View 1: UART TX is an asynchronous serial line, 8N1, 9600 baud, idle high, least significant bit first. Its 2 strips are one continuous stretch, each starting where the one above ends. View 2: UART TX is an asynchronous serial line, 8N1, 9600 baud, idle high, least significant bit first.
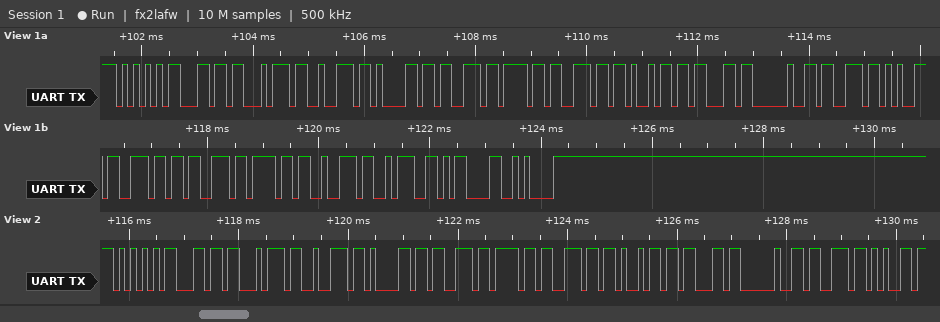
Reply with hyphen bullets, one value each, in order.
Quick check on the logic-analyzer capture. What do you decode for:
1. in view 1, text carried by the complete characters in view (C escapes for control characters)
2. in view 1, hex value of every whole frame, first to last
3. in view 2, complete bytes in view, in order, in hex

- "Ultrasonic sensor:\r\n"
- 55 6C 74 72 61 73 6F 6E 69 63 20 73 65 6E 73 6F 72 3A 0D 0A
- 0x55 0x6C 0x74 0x72 0x61 0x73 0x6F 0x6E 0x69 0x63 0x20 0x73 0x65
